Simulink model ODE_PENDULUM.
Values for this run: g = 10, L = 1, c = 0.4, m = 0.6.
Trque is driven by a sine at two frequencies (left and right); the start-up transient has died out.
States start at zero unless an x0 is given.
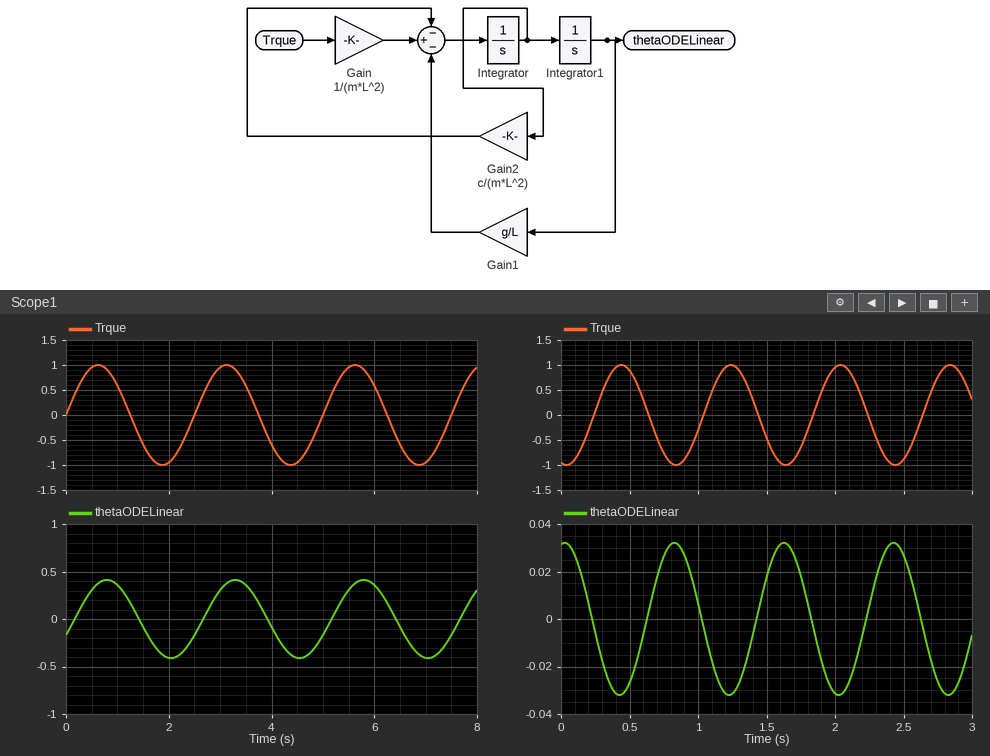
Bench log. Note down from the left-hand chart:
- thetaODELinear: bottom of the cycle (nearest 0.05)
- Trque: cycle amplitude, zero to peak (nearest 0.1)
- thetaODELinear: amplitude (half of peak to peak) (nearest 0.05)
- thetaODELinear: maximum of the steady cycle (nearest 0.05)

-0.40
1.0
0.40
0.40
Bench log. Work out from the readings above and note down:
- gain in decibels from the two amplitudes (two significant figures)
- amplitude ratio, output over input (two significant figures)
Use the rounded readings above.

-8.0 dB
0.40
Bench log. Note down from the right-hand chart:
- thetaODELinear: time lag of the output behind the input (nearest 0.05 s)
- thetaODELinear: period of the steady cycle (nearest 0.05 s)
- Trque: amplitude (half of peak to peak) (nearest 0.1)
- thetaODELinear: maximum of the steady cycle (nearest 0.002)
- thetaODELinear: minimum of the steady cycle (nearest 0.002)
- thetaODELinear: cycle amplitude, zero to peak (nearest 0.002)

0.40 s
0.80 s
1.0
0.032
-0.032
0.032
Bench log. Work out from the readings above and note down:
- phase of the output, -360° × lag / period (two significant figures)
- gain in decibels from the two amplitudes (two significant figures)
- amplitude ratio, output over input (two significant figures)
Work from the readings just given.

-180°
-30 dB
0.032
